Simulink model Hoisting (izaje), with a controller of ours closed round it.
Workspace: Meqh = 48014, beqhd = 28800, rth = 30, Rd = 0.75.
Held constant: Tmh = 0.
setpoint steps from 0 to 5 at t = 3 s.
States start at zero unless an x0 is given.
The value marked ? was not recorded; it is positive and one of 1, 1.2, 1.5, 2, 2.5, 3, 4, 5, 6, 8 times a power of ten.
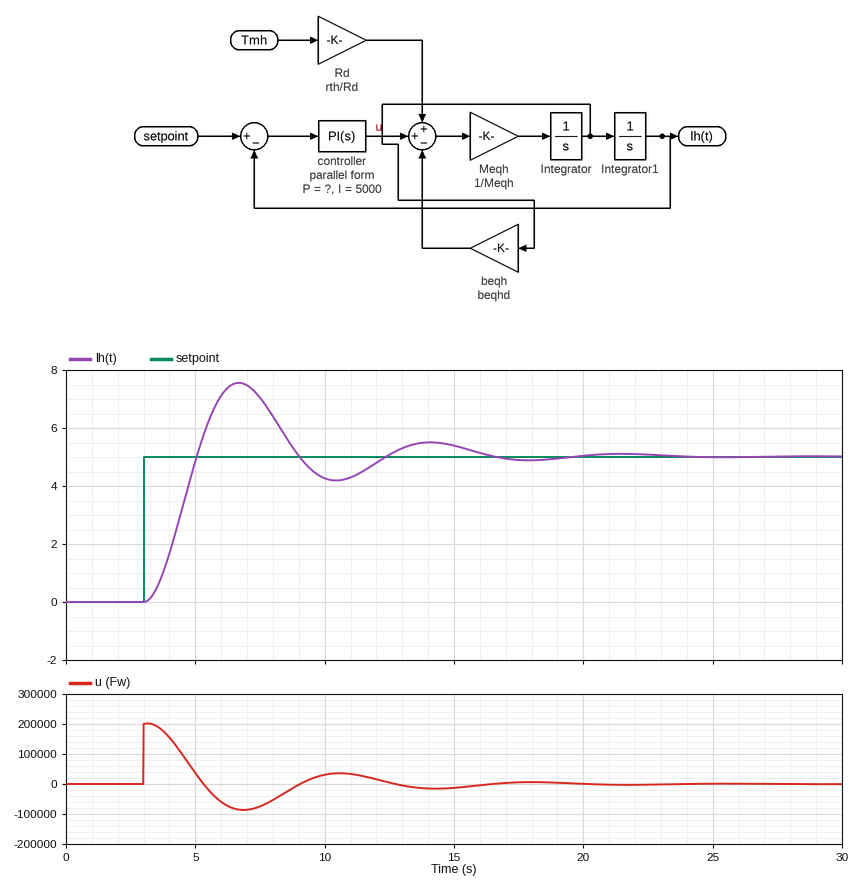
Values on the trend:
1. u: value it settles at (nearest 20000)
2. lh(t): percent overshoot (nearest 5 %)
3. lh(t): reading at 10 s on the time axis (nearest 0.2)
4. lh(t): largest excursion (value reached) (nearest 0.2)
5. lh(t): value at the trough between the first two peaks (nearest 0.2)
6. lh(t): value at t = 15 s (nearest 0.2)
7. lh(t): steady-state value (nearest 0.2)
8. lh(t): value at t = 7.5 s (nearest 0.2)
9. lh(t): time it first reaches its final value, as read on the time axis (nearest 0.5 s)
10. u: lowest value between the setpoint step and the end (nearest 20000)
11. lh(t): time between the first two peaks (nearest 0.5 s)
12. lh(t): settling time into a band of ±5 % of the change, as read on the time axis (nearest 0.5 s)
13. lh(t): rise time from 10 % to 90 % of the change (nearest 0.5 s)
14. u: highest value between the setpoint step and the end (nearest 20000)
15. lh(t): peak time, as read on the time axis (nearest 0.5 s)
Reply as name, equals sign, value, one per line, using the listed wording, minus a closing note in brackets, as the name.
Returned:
u: value it settles at = 0
lh(t): percent overshoot = 50 %
lh(t): reading at 10 s on the time axis = 4.2
lh(t): largest excursion (value reached) = 7.6
lh(t): value at the trough between the first two peaks = 4.2
lh(t): value at t = 15 s = 5.4
lh(t): steady-state value = 5.0
lh(t): value at t = 7.5 s = 7.0
lh(t): time it first reaches its final value, as read on the time axis = 5.0 s
u: lowest value between the setpoint step and the end = -80000
lh(t): time between the first two peaks = 7.5 s
lh(t): settling time into a band of ±5 % of the change, as read on the time axis = 15.5 s
lh(t): rise time from 10 % to 90 % of the change = 1.5 s
u: highest value between the setpoint step and the end = 200000
lh(t): peak time, as read on the time axis = 6.5 s
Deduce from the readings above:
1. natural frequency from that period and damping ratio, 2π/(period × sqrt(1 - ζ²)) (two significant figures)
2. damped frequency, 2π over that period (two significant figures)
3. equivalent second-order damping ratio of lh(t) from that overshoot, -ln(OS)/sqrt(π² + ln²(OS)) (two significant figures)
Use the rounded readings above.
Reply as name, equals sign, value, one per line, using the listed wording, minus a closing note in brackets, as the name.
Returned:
natural frequency from that period and damping ratio, 2π/(period × sqrt(1 - ζ²)) = 0.86 rad/s
damped frequency, 2π over that period = 0.84 rad/s
equivalent second-order damping ratio of lh(t) from that overshoot, -ln(OS)/sqrt(π² + ln²(OS)) = 0.22
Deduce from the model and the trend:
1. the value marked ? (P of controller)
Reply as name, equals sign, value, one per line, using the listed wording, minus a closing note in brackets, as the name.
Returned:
the value marked ? = 40000
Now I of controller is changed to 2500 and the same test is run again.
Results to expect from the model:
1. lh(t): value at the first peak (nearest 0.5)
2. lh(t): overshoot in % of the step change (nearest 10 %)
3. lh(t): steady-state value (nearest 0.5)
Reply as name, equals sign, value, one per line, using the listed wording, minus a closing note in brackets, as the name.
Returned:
lh(t): value at the first peak = 7.0
lh(t): overshoot in % of the step change = 40 %
lh(t): steady-state value = 5.0
